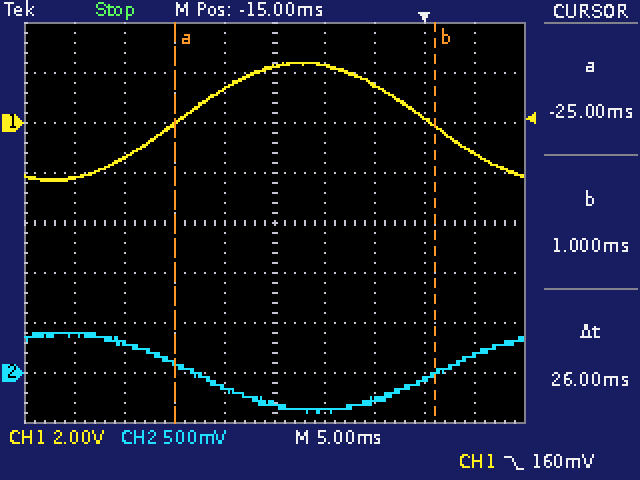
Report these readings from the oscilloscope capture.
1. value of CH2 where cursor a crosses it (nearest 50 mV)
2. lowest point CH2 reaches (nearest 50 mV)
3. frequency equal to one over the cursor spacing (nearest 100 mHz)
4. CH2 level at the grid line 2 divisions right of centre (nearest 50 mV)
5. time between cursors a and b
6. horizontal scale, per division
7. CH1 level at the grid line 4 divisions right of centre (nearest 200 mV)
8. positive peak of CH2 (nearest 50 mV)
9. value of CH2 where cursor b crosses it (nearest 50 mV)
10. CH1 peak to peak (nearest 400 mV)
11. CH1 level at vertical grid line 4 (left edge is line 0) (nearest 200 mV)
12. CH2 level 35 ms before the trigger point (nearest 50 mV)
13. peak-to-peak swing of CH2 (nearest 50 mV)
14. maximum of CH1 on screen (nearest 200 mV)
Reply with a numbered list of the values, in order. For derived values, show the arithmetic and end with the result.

1. 100 mV
2. -400 mV
3. 1 / 26 ms ≈ 38.5 Hz
4. -300 mV
5. 26 ms
6. 5 ms
7. -1.2 V
8. 400 mV
9. 0 mV
10. 4.8 V
11. 1.4 V
12. 400 mV
13. 400 mV − (-400 mV) = 800 mV
14. 2.4 V
